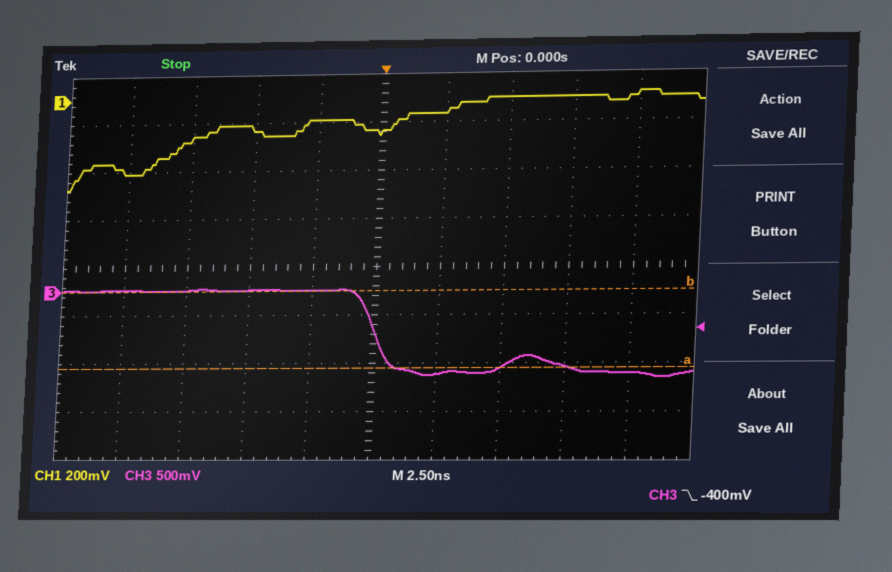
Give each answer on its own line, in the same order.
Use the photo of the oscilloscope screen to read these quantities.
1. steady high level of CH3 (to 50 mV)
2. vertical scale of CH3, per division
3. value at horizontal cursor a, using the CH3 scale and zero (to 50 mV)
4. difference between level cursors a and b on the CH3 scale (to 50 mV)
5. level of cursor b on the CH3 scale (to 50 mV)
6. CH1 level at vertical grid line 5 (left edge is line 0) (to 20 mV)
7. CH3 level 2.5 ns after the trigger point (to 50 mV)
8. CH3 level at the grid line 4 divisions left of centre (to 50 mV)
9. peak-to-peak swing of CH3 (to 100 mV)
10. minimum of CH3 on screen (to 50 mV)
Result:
0 mV
500 mV
-800 mV
800 mV
0 mV
-140 mV
-850 mV
0 mV
900 mV
-900 mV
